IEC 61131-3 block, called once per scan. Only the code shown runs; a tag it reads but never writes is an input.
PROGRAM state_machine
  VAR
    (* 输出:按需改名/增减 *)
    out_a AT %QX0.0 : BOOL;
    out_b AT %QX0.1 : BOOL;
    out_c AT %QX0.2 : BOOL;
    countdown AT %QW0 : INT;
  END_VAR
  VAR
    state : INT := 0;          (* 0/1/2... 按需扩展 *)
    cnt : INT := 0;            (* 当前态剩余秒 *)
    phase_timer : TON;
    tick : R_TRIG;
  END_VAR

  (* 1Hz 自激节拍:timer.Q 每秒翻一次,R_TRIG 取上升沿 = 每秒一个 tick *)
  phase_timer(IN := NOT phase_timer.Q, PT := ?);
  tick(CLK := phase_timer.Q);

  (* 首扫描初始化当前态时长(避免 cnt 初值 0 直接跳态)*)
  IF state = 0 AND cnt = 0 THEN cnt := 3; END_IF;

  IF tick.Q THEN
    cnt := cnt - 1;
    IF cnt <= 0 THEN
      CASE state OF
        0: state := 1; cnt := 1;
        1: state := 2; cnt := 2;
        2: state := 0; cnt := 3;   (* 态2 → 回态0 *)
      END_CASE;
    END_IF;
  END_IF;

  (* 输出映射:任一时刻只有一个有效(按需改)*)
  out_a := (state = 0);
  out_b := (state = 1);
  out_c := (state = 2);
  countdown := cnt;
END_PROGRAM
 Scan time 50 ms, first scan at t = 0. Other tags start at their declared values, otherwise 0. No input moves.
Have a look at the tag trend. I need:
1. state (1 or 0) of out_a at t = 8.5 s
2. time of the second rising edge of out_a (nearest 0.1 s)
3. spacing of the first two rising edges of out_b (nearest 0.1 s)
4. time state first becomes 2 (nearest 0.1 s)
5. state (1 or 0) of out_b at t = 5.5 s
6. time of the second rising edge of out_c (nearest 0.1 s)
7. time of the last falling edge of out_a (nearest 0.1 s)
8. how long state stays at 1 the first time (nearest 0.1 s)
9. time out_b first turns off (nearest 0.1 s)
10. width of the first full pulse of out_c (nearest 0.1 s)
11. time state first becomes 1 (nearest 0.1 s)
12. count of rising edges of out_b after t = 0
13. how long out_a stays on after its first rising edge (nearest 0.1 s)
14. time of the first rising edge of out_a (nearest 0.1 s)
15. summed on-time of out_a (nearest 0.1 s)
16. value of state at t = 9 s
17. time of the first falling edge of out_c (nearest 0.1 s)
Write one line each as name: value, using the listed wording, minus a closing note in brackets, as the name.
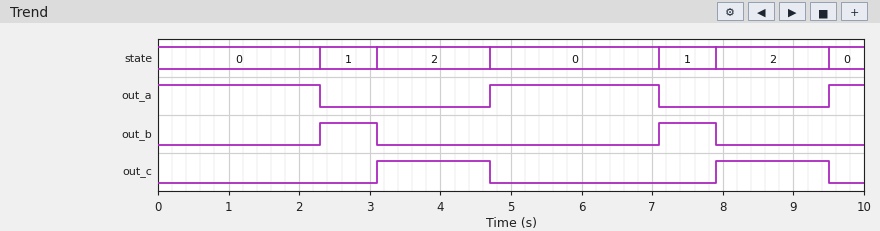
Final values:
state (1 or 0) of out_a at t = 8.5 s: 0
time of the second rising edge of out_a: 9.5 s
spacing of the first two rising edges of out_b: 4.8 s
time state first becomes 2: 3.1 s
state (1 or 0) of out_b at t = 5.5 s: 0
time of the second rising edge of out_c: 7.9 s
time of the last falling edge of out_a: 7.1 s
how long state stays at 1 the first time: 0.8 s
time out_b first turns off: 3.1 s
width of the first full pulse of out_c: 1.6 s
time state first becomes 1: 2.3 s
count of rising edges of out_b after t = 0: 2
how long out_a stays on after its first rising edge: 2.4 s
time of the first rising edge of out_a: 4.7 s
summed on-time of out_a: 5.2 s
value of state at t = 9 s: 2
time of the first falling edge of out_c: 4.7 s
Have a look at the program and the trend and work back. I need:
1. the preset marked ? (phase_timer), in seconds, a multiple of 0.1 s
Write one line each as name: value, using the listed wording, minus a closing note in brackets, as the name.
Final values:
the preset marked ? (phase_timer), in seconds, a multiple of 0.1 s: 0.7 s
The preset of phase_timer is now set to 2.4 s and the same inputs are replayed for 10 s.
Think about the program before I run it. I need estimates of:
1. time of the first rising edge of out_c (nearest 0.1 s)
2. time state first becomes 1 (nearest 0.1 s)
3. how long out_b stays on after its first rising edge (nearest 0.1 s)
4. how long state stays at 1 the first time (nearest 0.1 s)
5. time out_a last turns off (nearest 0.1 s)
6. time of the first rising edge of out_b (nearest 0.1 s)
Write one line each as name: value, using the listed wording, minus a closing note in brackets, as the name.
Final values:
time of the first rising edge of out_c: 9.9 s
time state first becomes 1: 7.4 s
how long out_b stays on after its first rising edge: 2.5 s
how long state stays at 1 the first time: 2.5 s
time out_a last turns off: 7.4 s
time of the first rising edge of out_b: 7.4 s
